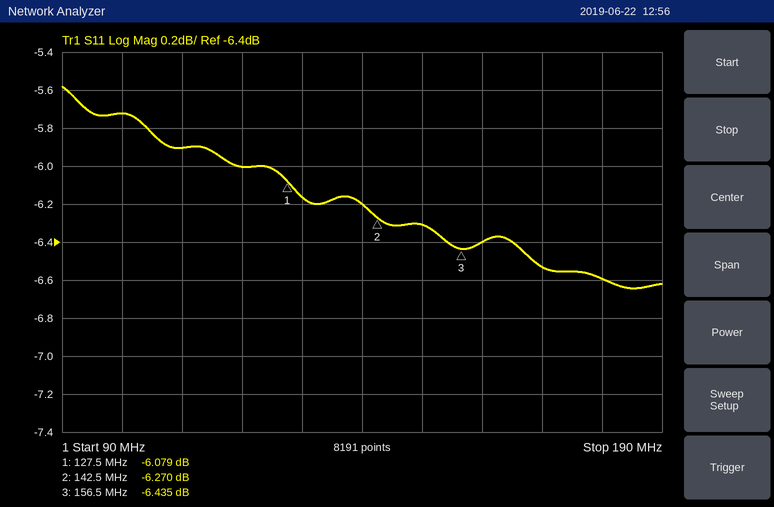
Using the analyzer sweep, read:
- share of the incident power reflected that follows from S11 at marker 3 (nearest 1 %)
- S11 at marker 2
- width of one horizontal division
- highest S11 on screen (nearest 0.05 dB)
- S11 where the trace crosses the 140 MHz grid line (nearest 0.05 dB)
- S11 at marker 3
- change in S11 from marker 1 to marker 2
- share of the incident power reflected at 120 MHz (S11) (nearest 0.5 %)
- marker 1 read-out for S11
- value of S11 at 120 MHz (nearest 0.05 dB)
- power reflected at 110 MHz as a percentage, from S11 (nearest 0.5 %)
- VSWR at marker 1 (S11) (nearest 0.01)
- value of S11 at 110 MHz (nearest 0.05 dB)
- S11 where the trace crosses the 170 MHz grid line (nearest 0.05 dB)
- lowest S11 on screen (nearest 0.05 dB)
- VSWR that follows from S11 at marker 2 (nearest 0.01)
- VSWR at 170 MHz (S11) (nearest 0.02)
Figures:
23 %
-6.270 dB
10 MHz
-5.60 dB
-6.20 dB
-6.435 dB
-0.191 dB
25.0 %
-6.079 dB
-6.00 dB
25.5 %
2.97
-5.90 dB
-6.55 dB
-6.65 dB
2.89
2.78
